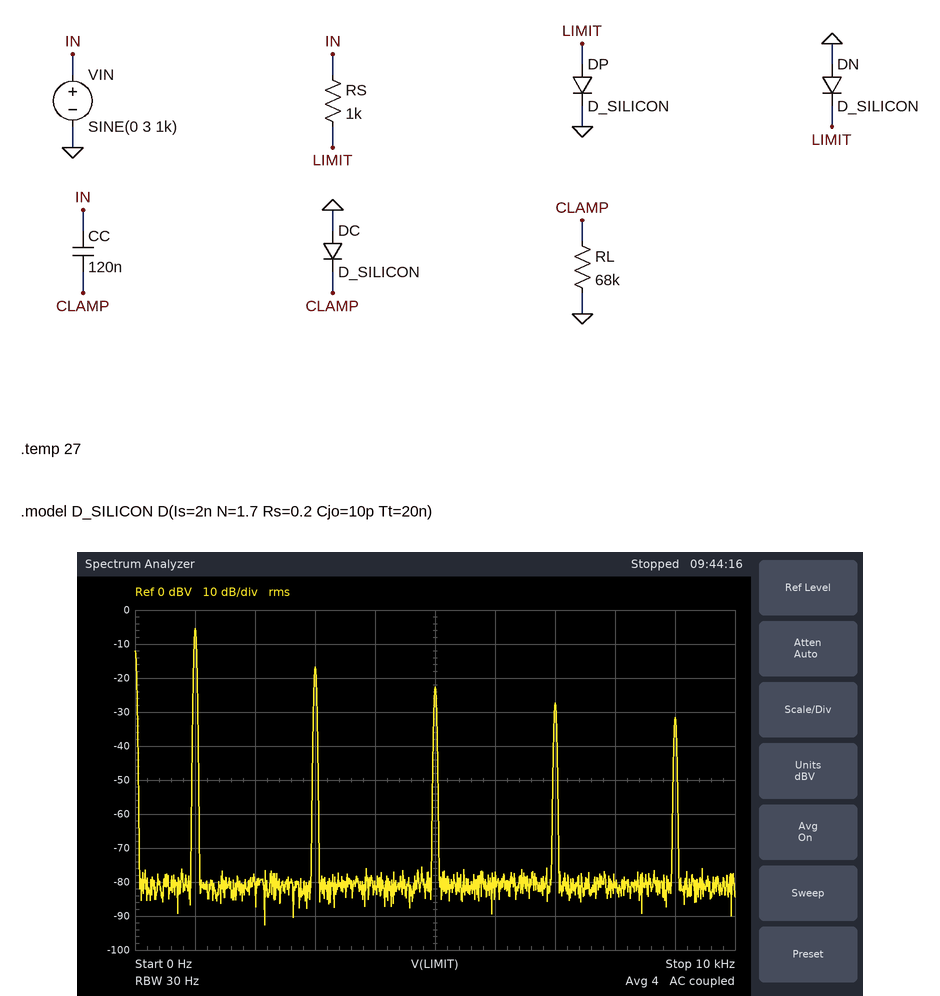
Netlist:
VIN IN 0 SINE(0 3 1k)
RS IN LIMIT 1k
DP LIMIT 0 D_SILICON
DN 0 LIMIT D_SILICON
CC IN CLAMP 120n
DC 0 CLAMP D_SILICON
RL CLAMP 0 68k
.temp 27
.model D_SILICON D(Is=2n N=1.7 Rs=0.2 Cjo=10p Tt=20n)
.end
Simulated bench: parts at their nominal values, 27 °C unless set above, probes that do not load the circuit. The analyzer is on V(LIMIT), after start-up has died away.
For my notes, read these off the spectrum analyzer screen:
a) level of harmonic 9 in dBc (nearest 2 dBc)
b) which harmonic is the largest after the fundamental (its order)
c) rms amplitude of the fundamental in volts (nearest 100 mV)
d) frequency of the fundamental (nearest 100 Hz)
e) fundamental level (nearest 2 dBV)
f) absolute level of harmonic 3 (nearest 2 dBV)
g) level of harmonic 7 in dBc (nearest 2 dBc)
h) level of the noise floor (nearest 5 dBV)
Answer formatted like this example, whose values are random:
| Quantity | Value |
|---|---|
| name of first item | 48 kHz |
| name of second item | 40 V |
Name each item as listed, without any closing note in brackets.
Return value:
| Quantity | Value |
|---|---|
| level of harmonic 9 in dBc | -26 dBc |
| which harmonic is the largest after the fundamental | 3 |
| rms amplitude of the fundamental in volts | 500 mV |
| frequency of the fundamental | 1.0 kHz |
| fundamental level | -6 dBV |
| absolute level of harmonic 3 | -16 dBV |
| level of harmonic 7 in dBc | -22 dBc |
| level of the noise floor | -80 dBV |
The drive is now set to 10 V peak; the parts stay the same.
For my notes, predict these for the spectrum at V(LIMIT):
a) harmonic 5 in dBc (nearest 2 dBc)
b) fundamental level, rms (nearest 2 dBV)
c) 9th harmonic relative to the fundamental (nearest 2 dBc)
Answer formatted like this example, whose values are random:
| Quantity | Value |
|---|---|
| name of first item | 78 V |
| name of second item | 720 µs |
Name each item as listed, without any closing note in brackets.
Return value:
| Quantity | Value |
|---|---|
| harmonic 5 in dBc | -16 dBc |
| fundamental level, rms | -4 dBV |
| 9th harmonic relative to the fundamental | -22 dBc |
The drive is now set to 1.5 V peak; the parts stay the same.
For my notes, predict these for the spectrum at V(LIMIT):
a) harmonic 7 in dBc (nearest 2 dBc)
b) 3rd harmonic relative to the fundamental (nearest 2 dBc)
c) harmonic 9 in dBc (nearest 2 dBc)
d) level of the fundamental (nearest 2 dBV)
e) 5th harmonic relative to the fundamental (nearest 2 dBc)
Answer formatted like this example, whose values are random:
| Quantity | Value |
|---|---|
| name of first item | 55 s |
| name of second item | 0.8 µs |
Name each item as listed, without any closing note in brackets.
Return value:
| Quantity | Value |
|---|---|
| harmonic 7 in dBc | -30 dBc |
| 3rd harmonic relative to the fundamental | -12 dBc |
| harmonic 9 in dBc | -44 dBc |
| level of the fundamental | -6 dBV |
| 5th harmonic relative to the fundamental | -22 dBc |
